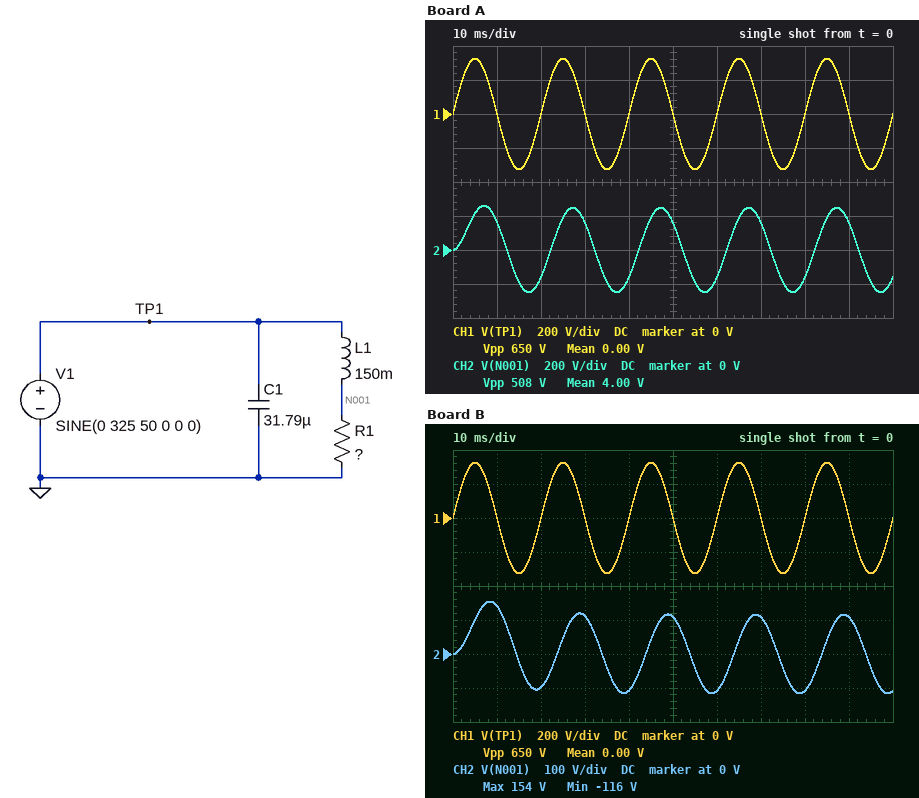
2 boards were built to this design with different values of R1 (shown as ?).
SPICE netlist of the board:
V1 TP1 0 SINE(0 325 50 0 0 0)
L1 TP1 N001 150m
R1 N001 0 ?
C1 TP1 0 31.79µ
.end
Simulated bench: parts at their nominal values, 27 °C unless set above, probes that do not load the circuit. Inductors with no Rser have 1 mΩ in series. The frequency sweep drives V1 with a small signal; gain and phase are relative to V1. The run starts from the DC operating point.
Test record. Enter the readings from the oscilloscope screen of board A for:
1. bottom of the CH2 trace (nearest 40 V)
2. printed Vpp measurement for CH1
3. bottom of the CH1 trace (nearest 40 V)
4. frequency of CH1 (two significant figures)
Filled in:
-240 V
650 V
-320 V
50 Hz
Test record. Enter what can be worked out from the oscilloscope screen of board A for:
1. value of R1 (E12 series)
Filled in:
56 Ω
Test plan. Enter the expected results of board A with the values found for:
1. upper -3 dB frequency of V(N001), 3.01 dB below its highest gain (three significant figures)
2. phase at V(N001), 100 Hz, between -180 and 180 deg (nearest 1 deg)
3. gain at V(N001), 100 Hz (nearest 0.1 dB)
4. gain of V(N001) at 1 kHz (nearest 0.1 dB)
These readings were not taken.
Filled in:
59.4 Hz
-59 deg
-5.8 dB
-24.5 dB
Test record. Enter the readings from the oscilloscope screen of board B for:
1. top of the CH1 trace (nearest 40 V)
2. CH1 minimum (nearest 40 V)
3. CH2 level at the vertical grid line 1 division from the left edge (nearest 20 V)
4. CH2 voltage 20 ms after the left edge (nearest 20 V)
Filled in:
320 V
-320 V
140 V
-100 V
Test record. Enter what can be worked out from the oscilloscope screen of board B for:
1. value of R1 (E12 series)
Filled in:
18 Ω
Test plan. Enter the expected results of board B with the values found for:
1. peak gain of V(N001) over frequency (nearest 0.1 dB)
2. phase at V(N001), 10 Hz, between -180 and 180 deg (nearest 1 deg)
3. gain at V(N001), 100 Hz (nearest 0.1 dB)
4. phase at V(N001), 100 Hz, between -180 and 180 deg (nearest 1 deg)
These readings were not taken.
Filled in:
0 dB
-28 deg
-14.5 dB
-79 deg
